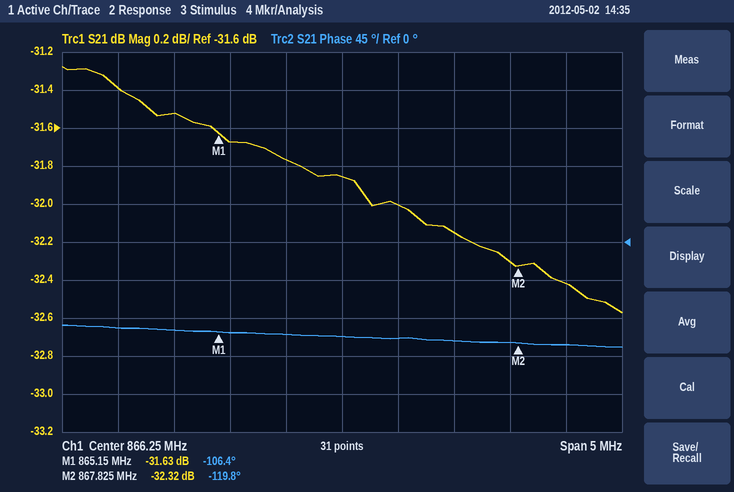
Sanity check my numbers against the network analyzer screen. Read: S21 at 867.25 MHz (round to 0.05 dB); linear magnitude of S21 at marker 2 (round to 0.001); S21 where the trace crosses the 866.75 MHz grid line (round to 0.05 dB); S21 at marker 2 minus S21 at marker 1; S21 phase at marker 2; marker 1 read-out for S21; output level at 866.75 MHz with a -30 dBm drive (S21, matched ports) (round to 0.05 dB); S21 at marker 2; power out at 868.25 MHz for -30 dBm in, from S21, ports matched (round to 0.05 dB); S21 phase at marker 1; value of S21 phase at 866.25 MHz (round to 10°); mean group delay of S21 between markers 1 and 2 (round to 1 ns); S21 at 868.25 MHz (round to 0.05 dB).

-32.15 dB
0.024
-32.00 dB
-0.69 dB
-119.8°
-31.63 dB
-62.00 dBm
-32.32 dB
-62.40 dBm
-106.4°
-110°
14 ns
-32.40 dB
